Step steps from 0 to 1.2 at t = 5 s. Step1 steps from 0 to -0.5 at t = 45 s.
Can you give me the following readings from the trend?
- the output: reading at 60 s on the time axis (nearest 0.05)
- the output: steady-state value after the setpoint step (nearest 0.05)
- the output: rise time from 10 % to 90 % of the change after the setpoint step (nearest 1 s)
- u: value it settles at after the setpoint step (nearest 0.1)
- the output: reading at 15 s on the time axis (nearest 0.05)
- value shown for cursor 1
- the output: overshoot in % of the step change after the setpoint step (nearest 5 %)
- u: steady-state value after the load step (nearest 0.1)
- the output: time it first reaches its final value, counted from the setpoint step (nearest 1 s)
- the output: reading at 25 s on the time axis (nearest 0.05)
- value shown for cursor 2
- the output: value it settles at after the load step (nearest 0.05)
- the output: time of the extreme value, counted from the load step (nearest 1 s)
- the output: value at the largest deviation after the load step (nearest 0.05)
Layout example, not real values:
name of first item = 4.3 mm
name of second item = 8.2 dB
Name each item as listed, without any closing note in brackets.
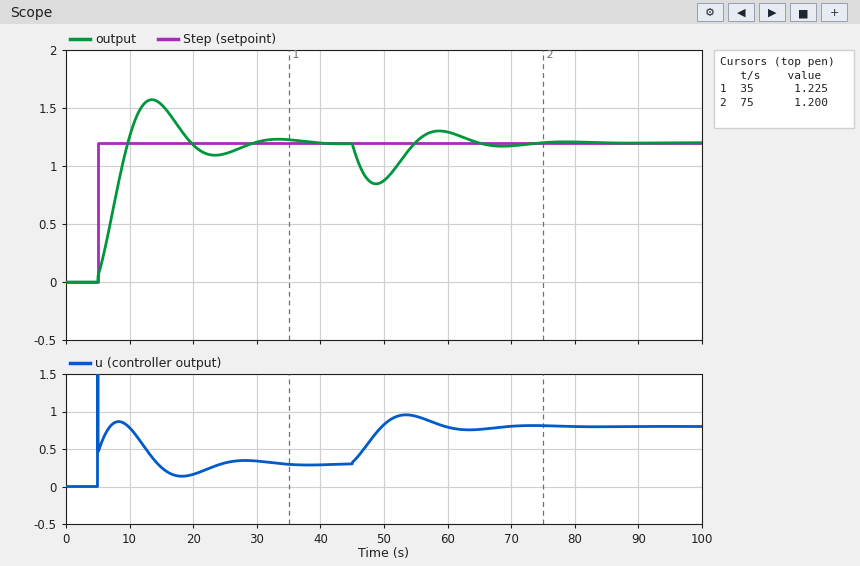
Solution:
the output: reading at 60 s on the time axis = 1.30
the output: steady-state value after the setpoint step = 1.20
the output: rise time from 10 % to 90 % of the change after the setpoint step = 4 s
u: value it settles at after the setpoint step = 0.3
the output: reading at 15 s on the time axis = 1.55
value shown for cursor 1 = 1.225
the output: overshoot in % of the step change after the setpoint step = 30 %
u: steady-state value after the load step = 0.8
the output: time it first reaches its final value, counted from the setpoint step = 5 s
the output: reading at 25 s on the time axis = 1.10
value shown for cursor 2 = 1.200
the output: value it settles at after the load step = 1.20
the output: time of the extreme value, counted from the load step = 4 s
the output: value at the largest deviation after the load step = 0.85
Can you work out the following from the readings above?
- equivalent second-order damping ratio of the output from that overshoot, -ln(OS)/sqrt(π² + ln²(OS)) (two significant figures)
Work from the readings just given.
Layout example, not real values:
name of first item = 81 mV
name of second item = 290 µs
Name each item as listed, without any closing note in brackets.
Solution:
equivalent second-order damping ratio of the output from that overshoot, -ln(OS)/sqrt(π² + ln²(OS)) = 0.36
